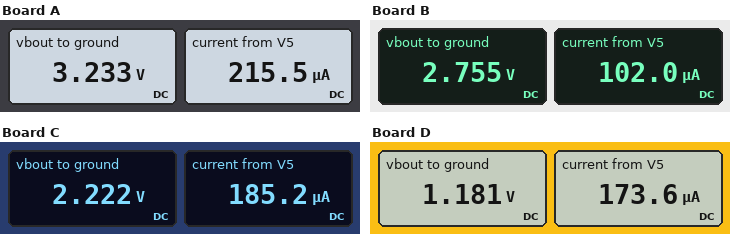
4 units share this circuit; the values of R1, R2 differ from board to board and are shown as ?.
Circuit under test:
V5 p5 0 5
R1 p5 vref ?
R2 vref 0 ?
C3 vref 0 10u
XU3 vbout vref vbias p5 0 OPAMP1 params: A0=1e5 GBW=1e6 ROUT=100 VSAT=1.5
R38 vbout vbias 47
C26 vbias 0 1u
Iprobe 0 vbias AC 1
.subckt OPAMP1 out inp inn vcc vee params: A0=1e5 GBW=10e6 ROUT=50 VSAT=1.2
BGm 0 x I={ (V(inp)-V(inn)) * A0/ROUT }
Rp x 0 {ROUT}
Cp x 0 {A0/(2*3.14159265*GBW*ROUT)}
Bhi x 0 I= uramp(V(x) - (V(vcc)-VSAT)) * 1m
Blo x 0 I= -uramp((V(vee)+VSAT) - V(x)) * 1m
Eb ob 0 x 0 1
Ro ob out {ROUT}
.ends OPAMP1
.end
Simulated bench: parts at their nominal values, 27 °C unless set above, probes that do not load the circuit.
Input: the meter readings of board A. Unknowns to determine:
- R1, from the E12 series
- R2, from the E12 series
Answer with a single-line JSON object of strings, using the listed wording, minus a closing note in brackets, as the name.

{"R1, from the E12 series": "8.2 kΩ", "R2, from the E12 series": "15 kΩ"}
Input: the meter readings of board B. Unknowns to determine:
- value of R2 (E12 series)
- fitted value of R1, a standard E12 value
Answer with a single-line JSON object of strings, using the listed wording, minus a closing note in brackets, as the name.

{"value of R2": "27 kΩ", "fitted value of R1, a standard E12 value": "22 kΩ"}
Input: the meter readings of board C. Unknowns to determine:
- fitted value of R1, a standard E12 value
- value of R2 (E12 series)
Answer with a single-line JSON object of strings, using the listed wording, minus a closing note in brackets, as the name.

{"fitted value of R1, a standard E12 value": "15 kΩ", "value of R2": "12 kΩ"}
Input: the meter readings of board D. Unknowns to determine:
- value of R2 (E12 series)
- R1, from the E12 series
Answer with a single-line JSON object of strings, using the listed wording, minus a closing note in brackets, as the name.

{"value of R2": "6.8 kΩ", "R1, from the E12 series": "22 kΩ"}
